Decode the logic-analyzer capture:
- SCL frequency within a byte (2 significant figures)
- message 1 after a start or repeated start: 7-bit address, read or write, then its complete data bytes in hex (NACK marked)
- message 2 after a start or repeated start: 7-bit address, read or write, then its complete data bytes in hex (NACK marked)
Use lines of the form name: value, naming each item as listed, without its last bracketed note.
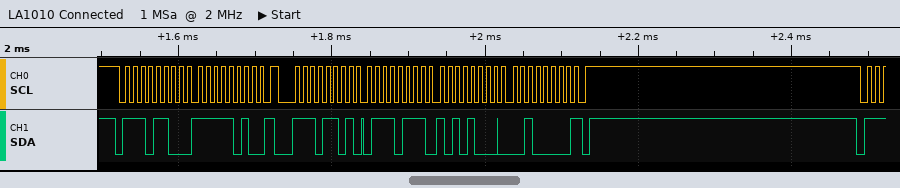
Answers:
SCL frequency within a byte: 100 kHz
message 1 after a start or repeated start: 7-bit address, read or write, then its complete data bytes in hex: 0x76 write: FA
message 2 after a start or repeated start: 7-bit address, read or write, then its complete data bytes in hex: 0x76 read: 77 A8 20 NACK
